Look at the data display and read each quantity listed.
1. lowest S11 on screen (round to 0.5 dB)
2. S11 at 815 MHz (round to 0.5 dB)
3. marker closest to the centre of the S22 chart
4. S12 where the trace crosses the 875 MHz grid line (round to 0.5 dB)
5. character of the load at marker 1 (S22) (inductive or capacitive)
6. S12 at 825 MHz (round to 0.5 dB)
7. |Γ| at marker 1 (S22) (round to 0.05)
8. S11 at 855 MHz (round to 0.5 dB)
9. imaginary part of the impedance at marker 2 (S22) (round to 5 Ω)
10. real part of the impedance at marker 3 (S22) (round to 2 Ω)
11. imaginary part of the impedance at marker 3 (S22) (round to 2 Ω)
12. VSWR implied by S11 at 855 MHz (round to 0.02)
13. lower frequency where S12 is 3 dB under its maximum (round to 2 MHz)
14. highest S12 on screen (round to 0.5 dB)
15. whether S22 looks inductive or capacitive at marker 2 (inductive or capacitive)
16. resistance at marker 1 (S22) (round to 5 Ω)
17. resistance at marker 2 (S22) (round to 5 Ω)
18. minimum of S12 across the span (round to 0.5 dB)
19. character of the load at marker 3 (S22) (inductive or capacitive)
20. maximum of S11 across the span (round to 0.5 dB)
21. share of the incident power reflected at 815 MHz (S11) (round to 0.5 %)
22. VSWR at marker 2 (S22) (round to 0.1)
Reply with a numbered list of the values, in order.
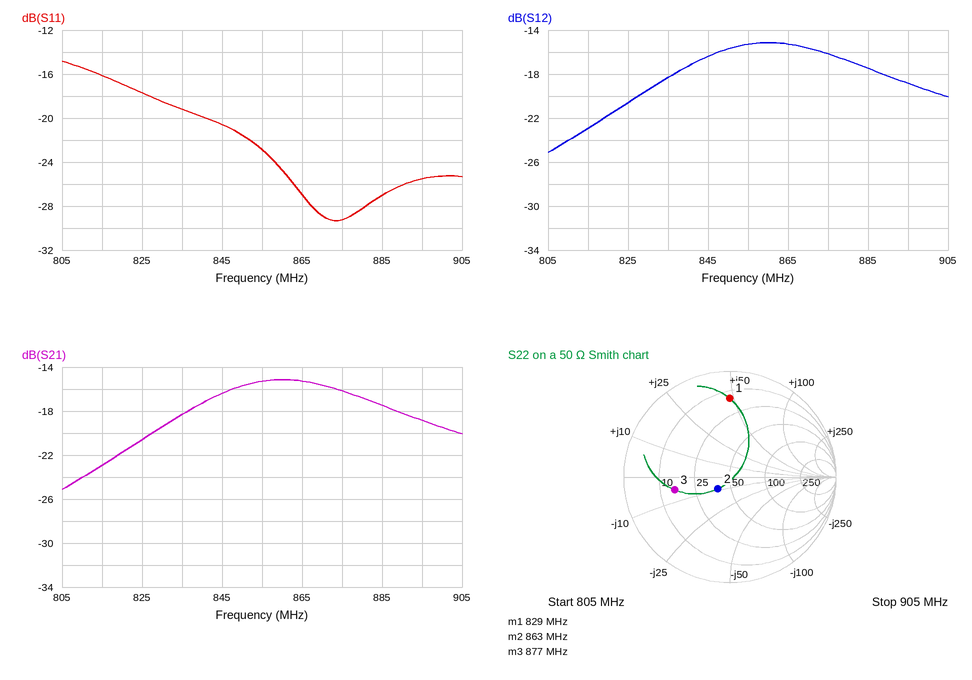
1. -29.5 dB
2. -16.0 dB
3. marker 2
4. -16.0 dB
5. inductive
6. -20.5 dB
7. 0.75
8. -23.0 dB
9. -10 Ω
10. 16 Ω
11. -6 Ω
12. 1.16
13. 836 MHz
14. -15.0 dB
15. capacitive
16. 15 Ω
17. 40 Ω
18. -25.0 dB
19. capacitive
20. -15.0 dB
21. 2.5 %
22. 1.4
